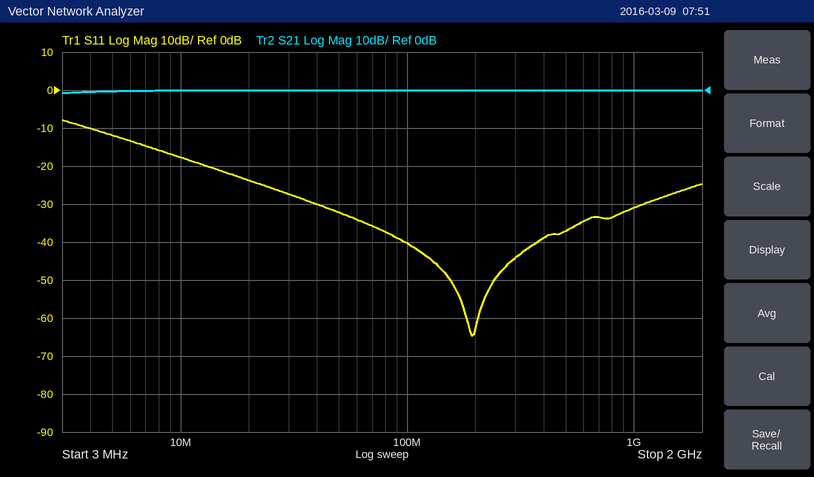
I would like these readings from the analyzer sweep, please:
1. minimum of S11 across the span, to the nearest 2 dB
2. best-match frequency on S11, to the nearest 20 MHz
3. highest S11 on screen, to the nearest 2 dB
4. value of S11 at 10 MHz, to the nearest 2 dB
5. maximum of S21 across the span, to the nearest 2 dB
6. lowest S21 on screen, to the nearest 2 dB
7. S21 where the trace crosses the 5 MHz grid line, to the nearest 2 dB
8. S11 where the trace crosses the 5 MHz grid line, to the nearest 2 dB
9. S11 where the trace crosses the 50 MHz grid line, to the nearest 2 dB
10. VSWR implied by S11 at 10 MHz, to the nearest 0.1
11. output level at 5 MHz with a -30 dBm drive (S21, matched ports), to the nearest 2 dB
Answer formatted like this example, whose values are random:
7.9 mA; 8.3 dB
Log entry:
-64 dB; 200 MHz; -8 dB; -18 dB; 0 dB; 0 dB; 0 dB; -12 dB; -32 dB; 1.3; -30 dBm
